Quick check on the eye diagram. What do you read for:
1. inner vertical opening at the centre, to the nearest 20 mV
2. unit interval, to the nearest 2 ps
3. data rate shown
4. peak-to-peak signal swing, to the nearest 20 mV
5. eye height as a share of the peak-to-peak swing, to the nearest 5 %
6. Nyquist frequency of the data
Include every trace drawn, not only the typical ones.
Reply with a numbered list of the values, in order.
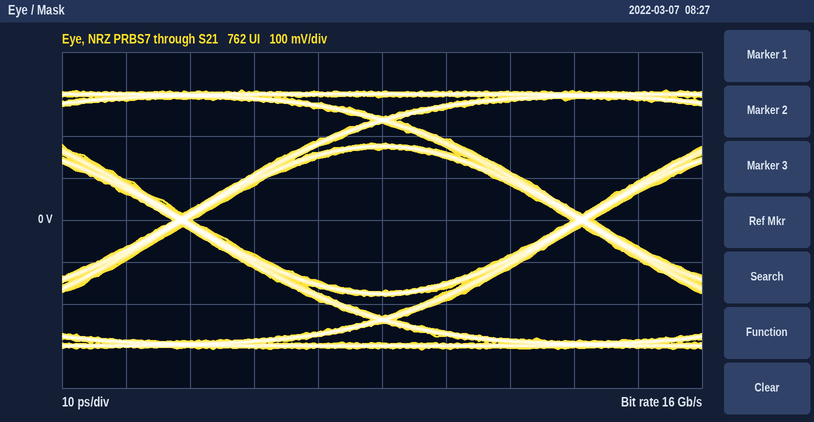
1. 340 mV
2. 62 ps
3. 16 Gb/s
4. 620 mV
5. 55 %
6. 8 GHz
